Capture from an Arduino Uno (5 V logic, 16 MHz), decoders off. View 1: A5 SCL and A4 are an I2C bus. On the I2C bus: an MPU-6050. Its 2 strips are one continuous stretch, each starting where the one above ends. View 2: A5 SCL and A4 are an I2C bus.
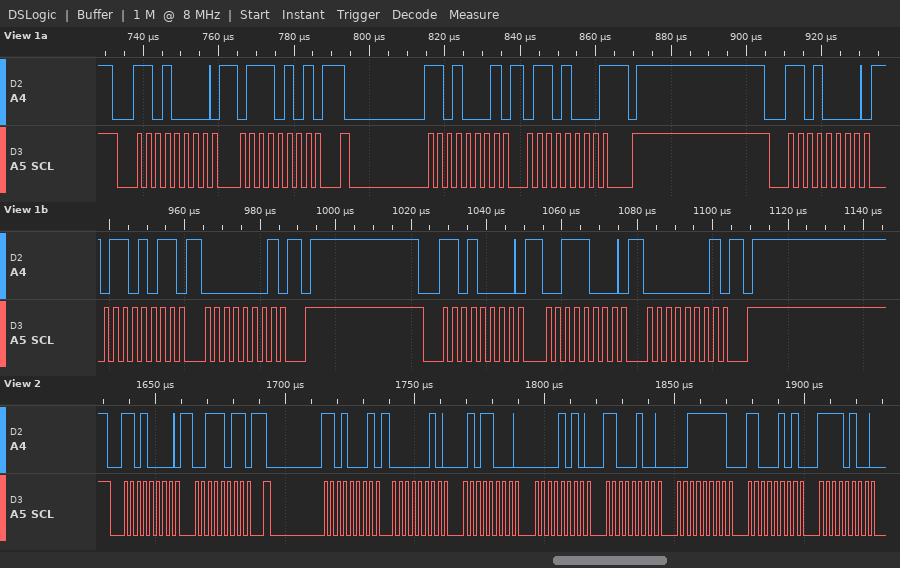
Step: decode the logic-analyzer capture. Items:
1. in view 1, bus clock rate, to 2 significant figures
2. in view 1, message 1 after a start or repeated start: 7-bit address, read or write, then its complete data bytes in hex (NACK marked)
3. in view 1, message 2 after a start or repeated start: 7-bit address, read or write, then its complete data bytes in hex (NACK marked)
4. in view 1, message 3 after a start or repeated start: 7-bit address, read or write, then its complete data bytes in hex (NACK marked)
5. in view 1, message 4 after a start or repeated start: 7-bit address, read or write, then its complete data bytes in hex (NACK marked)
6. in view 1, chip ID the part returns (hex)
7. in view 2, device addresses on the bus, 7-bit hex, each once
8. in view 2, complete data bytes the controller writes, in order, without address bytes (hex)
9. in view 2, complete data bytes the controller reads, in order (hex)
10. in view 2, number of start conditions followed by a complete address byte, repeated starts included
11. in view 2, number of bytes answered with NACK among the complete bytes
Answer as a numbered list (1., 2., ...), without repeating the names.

1. 400 kHz
2. 0x68 write: 75
3. 0x68 read: 68 NACK
4. 0x68 write: 6B 01
5. 0x68 write: 38 01
6. 0x68
7. 0x68
8. 3B
9. 02 58 0A C4 3F C5 F4
10. 2
11. 0
